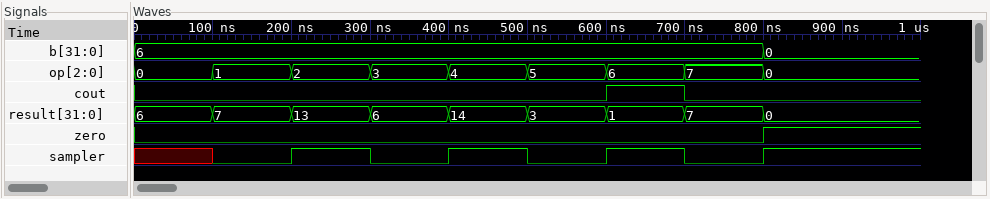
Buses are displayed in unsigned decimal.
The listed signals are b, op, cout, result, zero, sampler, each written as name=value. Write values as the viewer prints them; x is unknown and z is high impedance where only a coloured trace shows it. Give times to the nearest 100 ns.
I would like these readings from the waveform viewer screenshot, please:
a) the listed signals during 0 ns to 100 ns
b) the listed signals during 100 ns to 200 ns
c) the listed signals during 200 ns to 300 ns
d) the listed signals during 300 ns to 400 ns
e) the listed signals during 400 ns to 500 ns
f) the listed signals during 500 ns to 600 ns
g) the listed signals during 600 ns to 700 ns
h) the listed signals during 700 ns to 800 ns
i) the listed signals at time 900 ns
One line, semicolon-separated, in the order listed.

b=6, op=0, cout=0, result=6, zero=0, sampler=x; b=6, op=1, cout=0, result=7, zero=0, sampler=0; b=6, op=2, cout=0, result=13, zero=0, sampler=1; b=6, op=3, cout=0, result=6, zero=0, sampler=0; b=6, op=4, cout=0, result=14, zero=0, sampler=1; b=6, op=5, cout=0, result=3, zero=0, sampler=0; b=6, op=6, cout=1, result=1, zero=0, sampler=1; b=6, op=7, cout=0, result=7, zero=0, sampler=0; b=0, op=0, cout=0, result=0, zero=1, sampler=1
